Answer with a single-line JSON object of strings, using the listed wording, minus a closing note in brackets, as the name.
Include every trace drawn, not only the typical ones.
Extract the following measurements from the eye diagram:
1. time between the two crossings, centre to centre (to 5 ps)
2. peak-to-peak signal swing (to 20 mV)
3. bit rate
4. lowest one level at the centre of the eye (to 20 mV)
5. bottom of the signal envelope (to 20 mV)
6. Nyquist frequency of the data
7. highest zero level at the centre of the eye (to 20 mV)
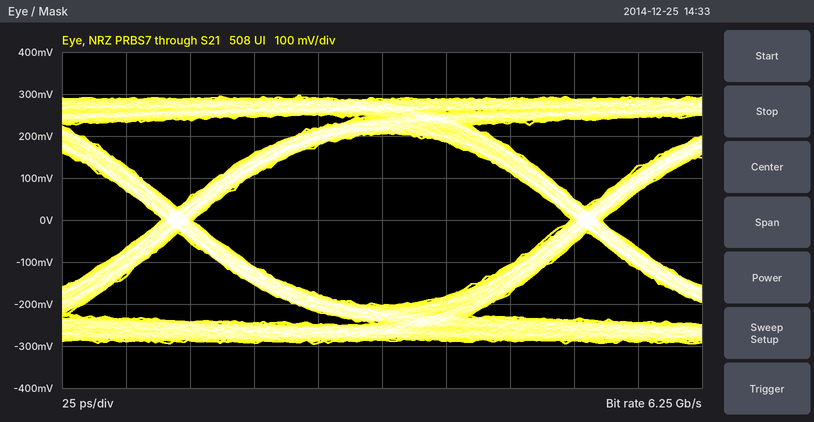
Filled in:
{"time between the two crossings, centre to centre": "160 ps", "peak-to-peak signal swing": "600 mV", "bit rate": "6.25 Gb/s", "lowest one level at the centre of the eye": "200 mV", "bottom of the signal envelope": "-300 mV", "Nyquist frequency of the data": "3.125 GHz", "highest zero level at the centre of the eye": "-200 mV"}
